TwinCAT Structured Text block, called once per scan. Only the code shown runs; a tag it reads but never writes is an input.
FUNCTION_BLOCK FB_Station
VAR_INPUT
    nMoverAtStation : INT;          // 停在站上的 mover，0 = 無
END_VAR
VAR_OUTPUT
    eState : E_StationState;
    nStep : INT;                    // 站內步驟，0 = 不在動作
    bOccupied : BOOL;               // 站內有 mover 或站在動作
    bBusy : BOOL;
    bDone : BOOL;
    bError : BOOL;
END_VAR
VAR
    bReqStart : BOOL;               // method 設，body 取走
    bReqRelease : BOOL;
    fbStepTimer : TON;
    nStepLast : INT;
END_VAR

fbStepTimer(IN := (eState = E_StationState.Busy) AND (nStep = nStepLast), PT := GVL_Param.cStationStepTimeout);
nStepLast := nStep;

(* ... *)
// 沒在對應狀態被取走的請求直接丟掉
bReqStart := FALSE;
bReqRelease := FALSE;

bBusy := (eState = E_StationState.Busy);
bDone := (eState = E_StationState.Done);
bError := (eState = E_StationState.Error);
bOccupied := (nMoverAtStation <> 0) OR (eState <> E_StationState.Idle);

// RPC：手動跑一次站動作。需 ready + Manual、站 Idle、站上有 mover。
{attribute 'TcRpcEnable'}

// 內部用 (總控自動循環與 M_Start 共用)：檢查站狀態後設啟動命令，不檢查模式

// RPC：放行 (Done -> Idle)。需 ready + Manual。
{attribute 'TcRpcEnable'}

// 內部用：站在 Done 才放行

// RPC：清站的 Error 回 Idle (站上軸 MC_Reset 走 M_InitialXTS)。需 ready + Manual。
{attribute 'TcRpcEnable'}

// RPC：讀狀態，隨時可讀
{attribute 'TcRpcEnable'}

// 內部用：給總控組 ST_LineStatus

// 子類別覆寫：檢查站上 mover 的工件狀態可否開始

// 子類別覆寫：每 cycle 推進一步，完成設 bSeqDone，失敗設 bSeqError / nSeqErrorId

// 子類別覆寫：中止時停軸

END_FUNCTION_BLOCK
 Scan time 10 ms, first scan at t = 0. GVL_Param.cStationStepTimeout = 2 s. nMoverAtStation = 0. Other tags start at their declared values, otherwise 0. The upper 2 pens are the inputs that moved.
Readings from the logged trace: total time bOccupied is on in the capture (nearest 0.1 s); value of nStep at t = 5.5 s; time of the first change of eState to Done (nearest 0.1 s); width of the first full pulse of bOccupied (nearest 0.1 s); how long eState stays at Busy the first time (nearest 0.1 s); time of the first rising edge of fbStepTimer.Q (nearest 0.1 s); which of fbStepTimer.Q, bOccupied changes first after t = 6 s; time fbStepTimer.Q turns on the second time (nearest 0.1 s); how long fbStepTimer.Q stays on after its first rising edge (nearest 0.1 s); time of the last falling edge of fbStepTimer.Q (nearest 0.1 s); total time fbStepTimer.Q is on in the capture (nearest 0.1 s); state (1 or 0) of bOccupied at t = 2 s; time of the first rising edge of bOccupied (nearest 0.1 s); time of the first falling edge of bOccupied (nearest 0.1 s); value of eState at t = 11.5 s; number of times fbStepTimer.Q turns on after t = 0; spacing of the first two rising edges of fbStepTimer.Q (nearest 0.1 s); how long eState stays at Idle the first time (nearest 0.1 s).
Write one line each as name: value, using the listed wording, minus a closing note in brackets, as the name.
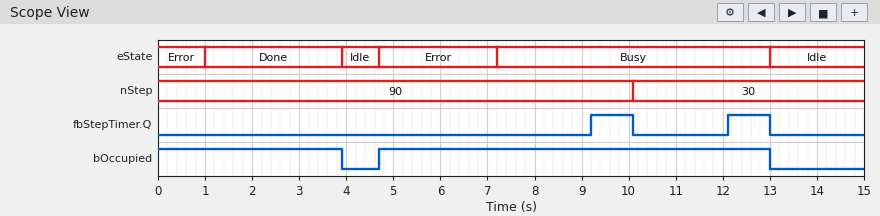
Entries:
total time bOccupied is on in the capture: 12.2 s
value of nStep at t = 5.5 s: 90
time of the first change of eState to Done: 1.0 s
width of the first full pulse of bOccupied: 8.3 s
how long eState stays at Busy the first time: 5.8 s
time of the first rising edge of fbStepTimer.Q: 9.2 s
which of fbStepTimer.Q, bOccupied changes first after t = 6 s: fbStepTimer.Q
time fbStepTimer.Q turns on the second time: 12.1 s
how long fbStepTimer.Q stays on after its first rising edge: 0.9 s
time of the last falling edge of fbStepTimer.Q: 13.0 s
total time fbStepTimer.Q is on in the capture: 1.8 s
state (1 or 0) of bOccupied at t = 2 s: 1
time of the first rising edge of bOccupied: 4.7 s
time of the first falling edge of bOccupied: 3.9 s
value of eState at t = 11.5 s: Busy
number of times fbStepTimer.Q turns on after t = 0: 2
spacing of the first two rising edges of fbStepTimer.Q: 2.9 s
how long eState stays at Idle the first time: 0.8 s
